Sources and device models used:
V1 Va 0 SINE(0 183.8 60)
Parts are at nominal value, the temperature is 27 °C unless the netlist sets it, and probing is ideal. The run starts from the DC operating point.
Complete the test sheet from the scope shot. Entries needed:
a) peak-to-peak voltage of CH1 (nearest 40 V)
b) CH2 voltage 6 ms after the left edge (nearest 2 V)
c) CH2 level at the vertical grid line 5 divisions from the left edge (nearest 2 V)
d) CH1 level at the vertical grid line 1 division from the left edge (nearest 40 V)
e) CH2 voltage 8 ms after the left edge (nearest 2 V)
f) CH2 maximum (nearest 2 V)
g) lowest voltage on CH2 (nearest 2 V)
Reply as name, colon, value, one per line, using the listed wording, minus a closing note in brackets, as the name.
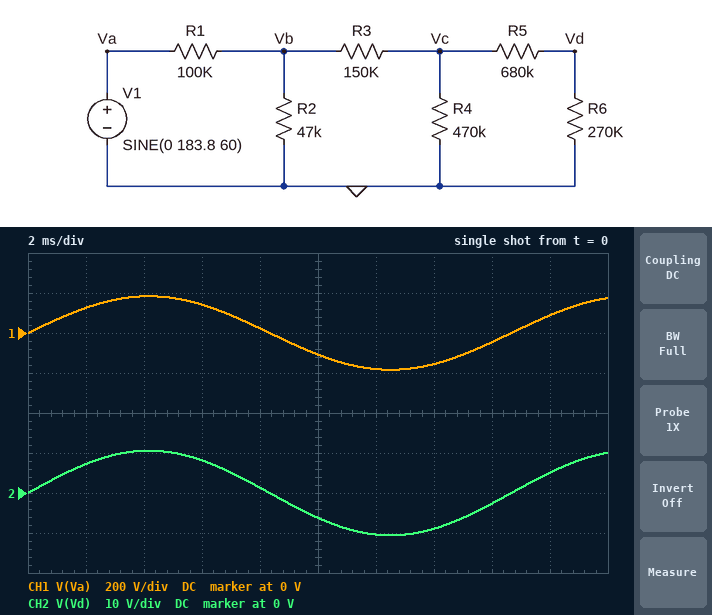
peak-to-peak voltage of CH1: 360 V
CH2 voltage 6 ms after the left edge: 8 V
CH2 level at the vertical grid line 5 divisions from the left edge: -6 V
CH1 level at the vertical grid line 1 division from the left edge: 120 V
CH2 voltage 8 ms after the left edge: 2 V
CH2 maximum: 10 V
lowest voltage on CH2: -10 V
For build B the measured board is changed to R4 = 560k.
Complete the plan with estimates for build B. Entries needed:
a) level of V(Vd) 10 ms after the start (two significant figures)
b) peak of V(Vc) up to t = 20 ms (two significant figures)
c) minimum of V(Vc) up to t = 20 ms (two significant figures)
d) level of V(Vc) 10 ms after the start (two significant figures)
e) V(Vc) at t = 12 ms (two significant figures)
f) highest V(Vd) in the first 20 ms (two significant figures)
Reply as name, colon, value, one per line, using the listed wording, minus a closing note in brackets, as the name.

level of V(Vd) 10 ms after the start: -6.5 V
peak of V(Vc) up to t = 20 ms: 39 V
minimum of V(Vc) up to t = 20 ms: -39 V
level of V(Vc) 10 ms after the start: -23 V
V(Vc) at t = 12 ms: -38 V
highest V(Vd) in the first 20 ms: 11 V
